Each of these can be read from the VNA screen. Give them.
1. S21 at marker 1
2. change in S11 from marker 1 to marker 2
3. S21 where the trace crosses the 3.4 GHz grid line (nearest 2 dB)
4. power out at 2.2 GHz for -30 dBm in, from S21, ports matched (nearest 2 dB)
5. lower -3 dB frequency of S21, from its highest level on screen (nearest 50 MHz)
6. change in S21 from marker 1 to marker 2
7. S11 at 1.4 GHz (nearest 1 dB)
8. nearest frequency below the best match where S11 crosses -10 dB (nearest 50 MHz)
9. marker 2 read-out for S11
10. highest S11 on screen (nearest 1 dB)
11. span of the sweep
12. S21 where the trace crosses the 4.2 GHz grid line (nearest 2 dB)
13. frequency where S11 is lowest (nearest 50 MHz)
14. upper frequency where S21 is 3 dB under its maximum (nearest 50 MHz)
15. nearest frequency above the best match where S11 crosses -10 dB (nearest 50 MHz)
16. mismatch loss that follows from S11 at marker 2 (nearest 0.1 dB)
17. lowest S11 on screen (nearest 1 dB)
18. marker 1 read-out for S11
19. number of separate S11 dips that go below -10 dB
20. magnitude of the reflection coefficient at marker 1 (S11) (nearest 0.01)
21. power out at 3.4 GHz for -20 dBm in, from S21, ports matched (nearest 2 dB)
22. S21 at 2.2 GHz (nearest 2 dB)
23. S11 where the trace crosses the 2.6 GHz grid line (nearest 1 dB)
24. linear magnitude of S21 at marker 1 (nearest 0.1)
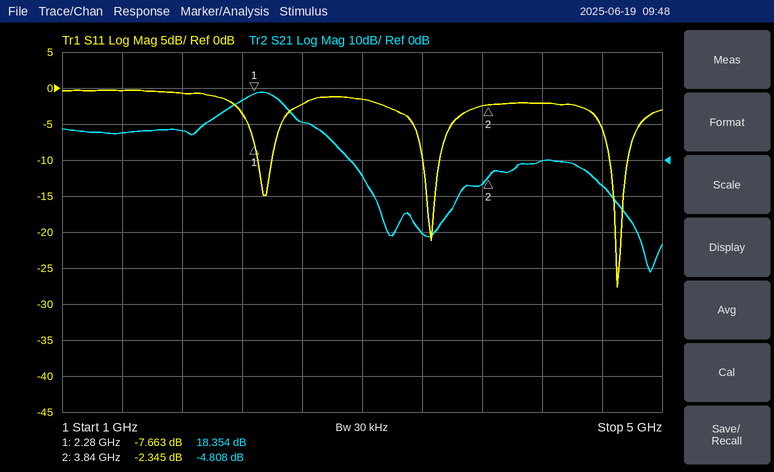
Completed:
18.354 dB
5.318 dB
-20 dB
-14 dBm
2.15 GHz
-23.162 dB
0 dB
4.65 GHz
-2.345 dB
0 dB
4 GHz
0 dB
4.70 GHz
2.45 GHz
4.75 GHz
3.8 dB
-28 dB
-7.663 dB
3
0.41
-40 dBm
16 dB
-2 dB
8.3
